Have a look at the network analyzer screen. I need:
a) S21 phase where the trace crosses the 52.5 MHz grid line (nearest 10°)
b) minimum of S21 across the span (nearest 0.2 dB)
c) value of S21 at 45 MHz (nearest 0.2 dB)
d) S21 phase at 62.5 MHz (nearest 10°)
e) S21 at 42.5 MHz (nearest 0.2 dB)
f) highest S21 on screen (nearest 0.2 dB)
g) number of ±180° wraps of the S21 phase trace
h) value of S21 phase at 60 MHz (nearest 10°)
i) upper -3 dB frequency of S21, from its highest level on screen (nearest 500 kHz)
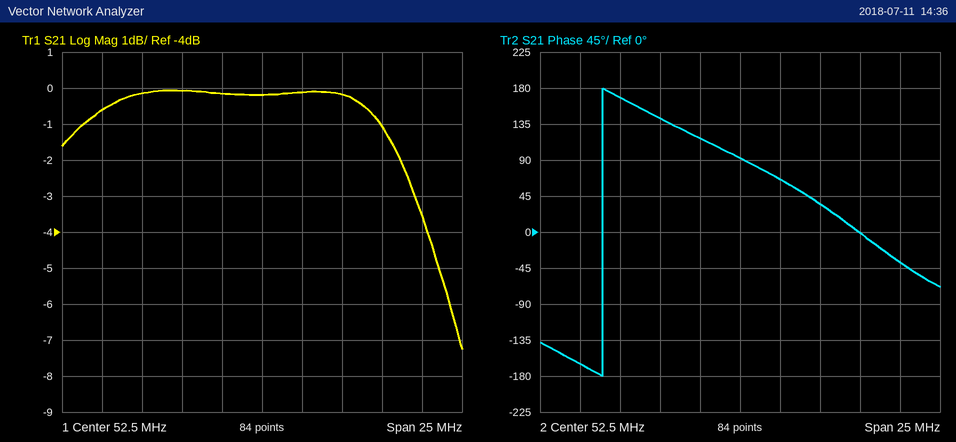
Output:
90°
-7.2 dB
-0.2 dB
-40°
-0.6 dB
0.0 dB
1
0°
62.0 MHz
